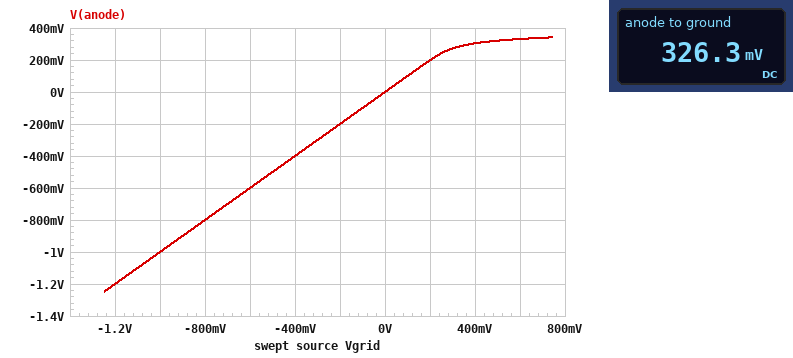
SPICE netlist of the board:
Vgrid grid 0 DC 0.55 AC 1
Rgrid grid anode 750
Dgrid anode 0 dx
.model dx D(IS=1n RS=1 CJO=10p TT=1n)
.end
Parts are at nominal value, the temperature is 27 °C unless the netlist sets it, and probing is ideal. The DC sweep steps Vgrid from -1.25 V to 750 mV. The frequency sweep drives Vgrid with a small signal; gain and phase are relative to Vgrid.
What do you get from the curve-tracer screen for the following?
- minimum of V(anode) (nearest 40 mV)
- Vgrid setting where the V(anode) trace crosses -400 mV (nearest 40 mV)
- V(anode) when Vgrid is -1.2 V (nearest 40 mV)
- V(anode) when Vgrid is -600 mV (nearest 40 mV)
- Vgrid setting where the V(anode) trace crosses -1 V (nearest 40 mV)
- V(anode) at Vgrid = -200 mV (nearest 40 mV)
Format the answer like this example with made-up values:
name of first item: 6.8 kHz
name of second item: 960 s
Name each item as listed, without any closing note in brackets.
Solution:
minimum of V(anode): -1.24 V
Vgrid setting where the V(anode) trace crosses -400 mV: -400 mV
V(anode) when Vgrid is -1.2 V: -1.20 V
V(anode) when Vgrid is -600 mV: -600 mV
Vgrid setting where the V(anode) trace crosses -1 V: -1.00 V
V(anode) at Vgrid = -200 mV: -200 mV
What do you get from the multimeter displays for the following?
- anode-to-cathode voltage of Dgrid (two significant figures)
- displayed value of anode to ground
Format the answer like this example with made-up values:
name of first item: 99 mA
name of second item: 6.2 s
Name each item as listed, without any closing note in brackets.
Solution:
anode-to-cathode voltage of Dgrid: 330 mV
displayed value of anode to ground: 326.3 mV
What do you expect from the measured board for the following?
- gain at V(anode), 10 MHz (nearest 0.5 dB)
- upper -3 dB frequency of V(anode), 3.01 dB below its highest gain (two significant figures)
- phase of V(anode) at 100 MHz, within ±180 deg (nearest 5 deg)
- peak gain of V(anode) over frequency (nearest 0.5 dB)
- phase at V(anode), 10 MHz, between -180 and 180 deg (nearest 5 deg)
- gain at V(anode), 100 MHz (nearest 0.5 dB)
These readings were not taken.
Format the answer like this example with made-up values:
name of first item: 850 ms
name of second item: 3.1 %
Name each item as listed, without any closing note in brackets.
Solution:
gain at V(anode), 10 MHz: -19.5 dB
upper -3 dB frequency of V(anode), 3.01 dB below its highest gain: 86 MHz
phase of V(anode) at 100 MHz, within ±180 deg: -50 deg
peak gain of V(anode) over frequency: -19.5 dB
phase at V(anode), 10 MHz, between -180 and 180 deg: -5 deg
gain at V(anode), 100 MHz: -23.5 dB
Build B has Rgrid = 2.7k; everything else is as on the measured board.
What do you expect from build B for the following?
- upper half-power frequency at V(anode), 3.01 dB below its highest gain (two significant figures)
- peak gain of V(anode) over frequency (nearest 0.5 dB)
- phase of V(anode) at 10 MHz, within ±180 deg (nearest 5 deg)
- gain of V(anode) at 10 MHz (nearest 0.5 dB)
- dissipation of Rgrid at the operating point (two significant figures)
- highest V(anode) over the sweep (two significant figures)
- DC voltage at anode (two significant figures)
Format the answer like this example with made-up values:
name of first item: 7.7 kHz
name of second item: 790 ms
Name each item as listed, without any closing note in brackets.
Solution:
upper half-power frequency at V(anode), 3.01 dB below its highest gain: 41 MHz
peak gain of V(anode) over frequency: -20.5 dB
phase of V(anode) at 10 MHz, within ±180 deg: -15 deg
gain of V(anode) at 10 MHz: -21.0 dB
dissipation of Rgrid at the operating point: 24 µW
highest V(anode) over the sweep: 310 mV
DC voltage at anode: 300 mV
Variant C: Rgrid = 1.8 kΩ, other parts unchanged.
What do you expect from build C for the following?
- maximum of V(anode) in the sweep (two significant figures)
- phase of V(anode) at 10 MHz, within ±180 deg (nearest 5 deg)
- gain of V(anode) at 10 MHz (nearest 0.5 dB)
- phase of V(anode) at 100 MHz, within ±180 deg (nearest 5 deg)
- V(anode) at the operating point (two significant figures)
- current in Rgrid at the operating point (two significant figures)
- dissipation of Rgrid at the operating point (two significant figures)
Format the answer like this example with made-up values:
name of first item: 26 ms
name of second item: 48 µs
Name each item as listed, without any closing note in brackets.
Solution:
maximum of V(anode) in the sweep: 320 mV
phase of V(anode) at 10 MHz, within ±180 deg: -10 deg
gain of V(anode) at 10 MHz: -20.5 dB
phase of V(anode) at 100 MHz, within ±180 deg: -60 deg
V(anode) at the operating point: 310 mV
current in Rgrid at the operating point: 140 µA
dissipation of Rgrid at the operating point: 33 µW
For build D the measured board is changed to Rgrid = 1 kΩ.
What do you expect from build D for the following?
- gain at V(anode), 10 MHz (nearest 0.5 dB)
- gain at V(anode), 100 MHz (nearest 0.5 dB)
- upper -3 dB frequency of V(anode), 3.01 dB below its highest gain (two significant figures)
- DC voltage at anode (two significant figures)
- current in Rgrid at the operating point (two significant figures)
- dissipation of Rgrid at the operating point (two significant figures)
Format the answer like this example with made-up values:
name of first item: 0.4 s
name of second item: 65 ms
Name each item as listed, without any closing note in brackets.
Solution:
gain at V(anode), 10 MHz: -20.0 dB
gain at V(anode), 100 MHz: -24.5 dB
upper -3 dB frequency of V(anode), 3.01 dB below its highest gain: 75 MHz
DC voltage at anode: 320 mV
current in Rgrid at the operating point: 230 µA
dissipation of Rgrid at the operating point: 53 µW
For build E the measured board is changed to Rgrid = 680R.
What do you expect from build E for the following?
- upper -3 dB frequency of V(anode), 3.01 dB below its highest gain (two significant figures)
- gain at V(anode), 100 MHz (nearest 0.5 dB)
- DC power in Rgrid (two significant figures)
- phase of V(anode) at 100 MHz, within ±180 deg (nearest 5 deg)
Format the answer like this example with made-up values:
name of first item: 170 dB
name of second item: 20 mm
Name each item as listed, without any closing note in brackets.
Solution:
upper -3 dB frequency of V(anode), 3.01 dB below its highest gain: 90 MHz
gain at V(anode), 100 MHz: -23.0 dB
DC power in Rgrid: 72 µW
phase of V(anode) at 100 MHz, within ±180 deg: -45 deg
